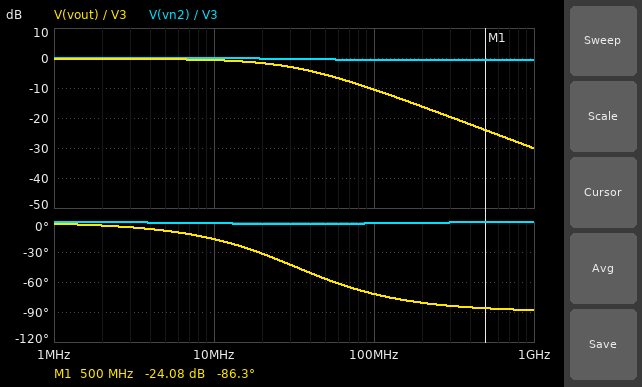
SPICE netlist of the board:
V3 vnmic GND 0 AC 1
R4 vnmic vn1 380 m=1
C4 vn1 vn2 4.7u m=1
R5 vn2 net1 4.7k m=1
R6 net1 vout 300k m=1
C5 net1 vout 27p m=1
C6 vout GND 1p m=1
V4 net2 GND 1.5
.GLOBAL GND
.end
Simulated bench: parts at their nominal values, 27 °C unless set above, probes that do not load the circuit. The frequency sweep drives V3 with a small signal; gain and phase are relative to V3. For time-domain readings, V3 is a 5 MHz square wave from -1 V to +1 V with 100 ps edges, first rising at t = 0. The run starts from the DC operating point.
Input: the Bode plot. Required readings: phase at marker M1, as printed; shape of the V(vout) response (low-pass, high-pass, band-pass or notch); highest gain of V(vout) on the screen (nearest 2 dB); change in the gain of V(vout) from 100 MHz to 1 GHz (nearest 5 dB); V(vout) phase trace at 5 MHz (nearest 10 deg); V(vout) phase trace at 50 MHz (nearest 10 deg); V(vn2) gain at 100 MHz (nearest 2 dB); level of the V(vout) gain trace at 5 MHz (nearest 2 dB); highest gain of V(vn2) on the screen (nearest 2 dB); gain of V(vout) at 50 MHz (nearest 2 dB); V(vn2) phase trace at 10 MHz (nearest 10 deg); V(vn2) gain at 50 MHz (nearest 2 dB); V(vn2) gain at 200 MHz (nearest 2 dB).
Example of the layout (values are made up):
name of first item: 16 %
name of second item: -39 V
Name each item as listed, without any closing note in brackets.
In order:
phase at marker M1, as printed: -86.3 deg
shape of the V(vout) response: low-pass
highest gain of V(vout) on the screen: 0 dB
change in the gain of V(vout) from 100 MHz to 1 GHz: -20 dB
V(vout) phase trace at 5 MHz: -10 deg
V(vout) phase trace at 50 MHz: -60 deg
V(vn2) gain at 100 MHz: 0 dB
level of the V(vout) gain trace at 5 MHz: 0 dB
highest gain of V(vn2) on the screen: 0 dB
gain of V(vout) at 50 MHz: -6 dB
V(vn2) phase trace at 10 MHz: 0 deg
V(vn2) gain at 50 MHz: 0 dB
V(vn2) gain at 200 MHz: 0 dB
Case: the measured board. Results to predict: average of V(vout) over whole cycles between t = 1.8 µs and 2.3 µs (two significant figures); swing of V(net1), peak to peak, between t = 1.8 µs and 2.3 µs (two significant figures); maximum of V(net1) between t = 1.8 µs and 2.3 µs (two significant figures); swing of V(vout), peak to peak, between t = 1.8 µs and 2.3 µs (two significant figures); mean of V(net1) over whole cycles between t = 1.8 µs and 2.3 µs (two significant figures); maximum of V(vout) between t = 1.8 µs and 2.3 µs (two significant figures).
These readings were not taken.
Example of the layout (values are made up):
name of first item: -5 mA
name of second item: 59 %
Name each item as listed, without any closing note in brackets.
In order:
average of V(vout) over whole cycles between t = 1.8 µs and 2.3 µs: 970 mV
swing of V(net1), peak to peak, between t = 1.8 µs and 2.3 µs: 2.0 V
maximum of V(net1) between t = 1.8 µs and 2.3 µs: 2.0 V
swing of V(vout), peak to peak, between t = 1.8 µs and 2.3 µs: 1.9 V
mean of V(net1) over whole cycles between t = 1.8 µs and 2.3 µs: 1.0 V
maximum of V(vout) between t = 1.8 µs and 2.3 µs: 1.9 V
